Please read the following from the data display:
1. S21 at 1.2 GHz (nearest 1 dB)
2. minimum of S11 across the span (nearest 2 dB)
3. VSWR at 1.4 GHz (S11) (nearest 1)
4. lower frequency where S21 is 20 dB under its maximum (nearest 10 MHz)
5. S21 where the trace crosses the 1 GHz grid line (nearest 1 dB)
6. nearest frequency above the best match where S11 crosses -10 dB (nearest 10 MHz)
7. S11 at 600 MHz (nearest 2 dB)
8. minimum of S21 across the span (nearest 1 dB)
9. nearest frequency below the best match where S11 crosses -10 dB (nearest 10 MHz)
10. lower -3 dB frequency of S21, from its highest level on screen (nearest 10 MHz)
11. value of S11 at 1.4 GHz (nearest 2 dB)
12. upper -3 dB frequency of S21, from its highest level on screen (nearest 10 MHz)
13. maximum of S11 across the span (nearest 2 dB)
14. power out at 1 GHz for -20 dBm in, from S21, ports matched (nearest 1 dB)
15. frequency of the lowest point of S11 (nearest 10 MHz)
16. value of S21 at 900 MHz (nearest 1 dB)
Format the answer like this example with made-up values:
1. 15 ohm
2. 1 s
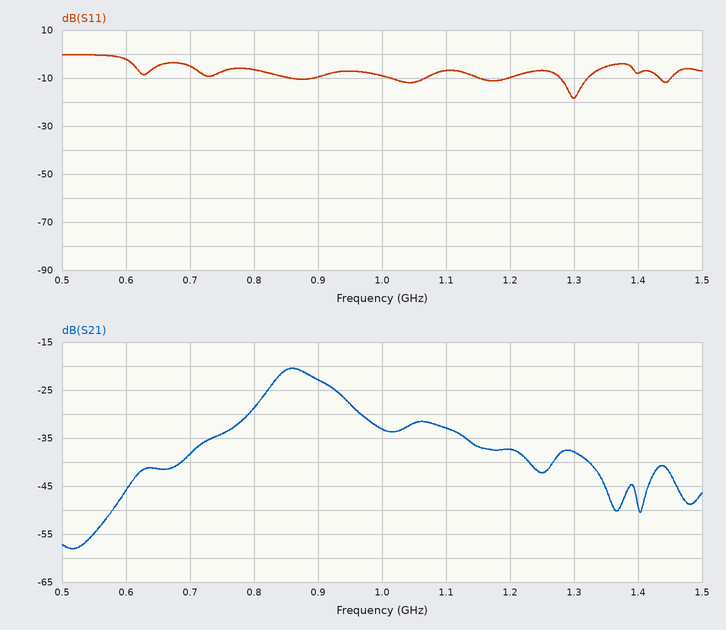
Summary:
1. -37 dB
2. -18 dB
3. 2
4. 680 MHz
5. -33 dB
6. 1.32 GHz
7. -2 dB
8. -58 dB
9. 1.28 GHz
10. 830 MHz
11. -8 dB
12. 910 MHz
13. 0 dB
14. -53 dBm
15. 1.30 GHz
16. -23 dB
